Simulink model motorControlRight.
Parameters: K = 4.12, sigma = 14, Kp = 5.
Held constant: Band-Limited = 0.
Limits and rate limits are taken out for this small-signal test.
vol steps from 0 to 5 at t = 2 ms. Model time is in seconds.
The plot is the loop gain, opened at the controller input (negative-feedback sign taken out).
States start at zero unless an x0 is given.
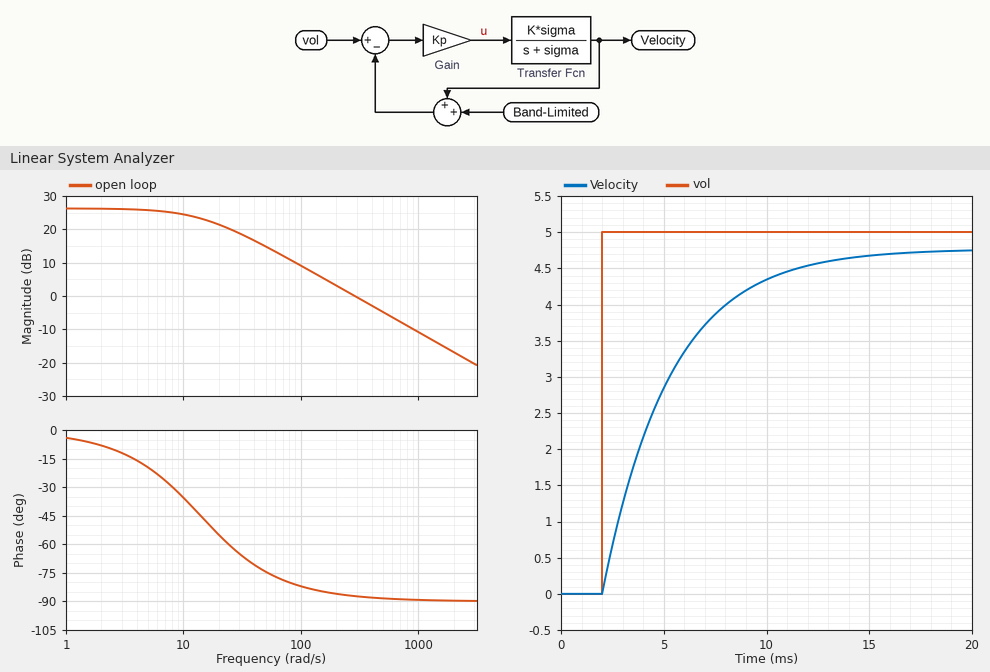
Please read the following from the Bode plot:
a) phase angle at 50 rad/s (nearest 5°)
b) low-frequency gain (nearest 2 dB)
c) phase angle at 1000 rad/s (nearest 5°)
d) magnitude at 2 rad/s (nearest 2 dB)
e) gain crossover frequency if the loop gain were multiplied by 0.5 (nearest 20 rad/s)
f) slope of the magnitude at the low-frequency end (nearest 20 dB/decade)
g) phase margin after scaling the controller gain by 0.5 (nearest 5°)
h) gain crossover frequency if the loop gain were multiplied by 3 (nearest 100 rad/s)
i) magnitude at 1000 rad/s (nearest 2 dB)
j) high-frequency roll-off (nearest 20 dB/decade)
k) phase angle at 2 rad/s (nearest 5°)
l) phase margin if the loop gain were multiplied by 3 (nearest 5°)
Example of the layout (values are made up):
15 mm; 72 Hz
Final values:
-75°; 26 dB; -90°; 26 dB; 140 rad/s; 0 dB/decade; 95°; 900 rad/s; -10 dB; -20 dB/decade; -10°; 90°
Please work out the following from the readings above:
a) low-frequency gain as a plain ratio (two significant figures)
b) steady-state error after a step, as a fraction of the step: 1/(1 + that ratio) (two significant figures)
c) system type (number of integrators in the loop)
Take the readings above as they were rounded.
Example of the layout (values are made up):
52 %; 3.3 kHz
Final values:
20; 0.048; 0
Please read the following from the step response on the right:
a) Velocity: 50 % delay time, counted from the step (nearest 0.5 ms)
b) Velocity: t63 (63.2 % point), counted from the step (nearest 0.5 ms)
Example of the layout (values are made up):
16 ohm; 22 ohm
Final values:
2.5 ms; 3.5 ms
